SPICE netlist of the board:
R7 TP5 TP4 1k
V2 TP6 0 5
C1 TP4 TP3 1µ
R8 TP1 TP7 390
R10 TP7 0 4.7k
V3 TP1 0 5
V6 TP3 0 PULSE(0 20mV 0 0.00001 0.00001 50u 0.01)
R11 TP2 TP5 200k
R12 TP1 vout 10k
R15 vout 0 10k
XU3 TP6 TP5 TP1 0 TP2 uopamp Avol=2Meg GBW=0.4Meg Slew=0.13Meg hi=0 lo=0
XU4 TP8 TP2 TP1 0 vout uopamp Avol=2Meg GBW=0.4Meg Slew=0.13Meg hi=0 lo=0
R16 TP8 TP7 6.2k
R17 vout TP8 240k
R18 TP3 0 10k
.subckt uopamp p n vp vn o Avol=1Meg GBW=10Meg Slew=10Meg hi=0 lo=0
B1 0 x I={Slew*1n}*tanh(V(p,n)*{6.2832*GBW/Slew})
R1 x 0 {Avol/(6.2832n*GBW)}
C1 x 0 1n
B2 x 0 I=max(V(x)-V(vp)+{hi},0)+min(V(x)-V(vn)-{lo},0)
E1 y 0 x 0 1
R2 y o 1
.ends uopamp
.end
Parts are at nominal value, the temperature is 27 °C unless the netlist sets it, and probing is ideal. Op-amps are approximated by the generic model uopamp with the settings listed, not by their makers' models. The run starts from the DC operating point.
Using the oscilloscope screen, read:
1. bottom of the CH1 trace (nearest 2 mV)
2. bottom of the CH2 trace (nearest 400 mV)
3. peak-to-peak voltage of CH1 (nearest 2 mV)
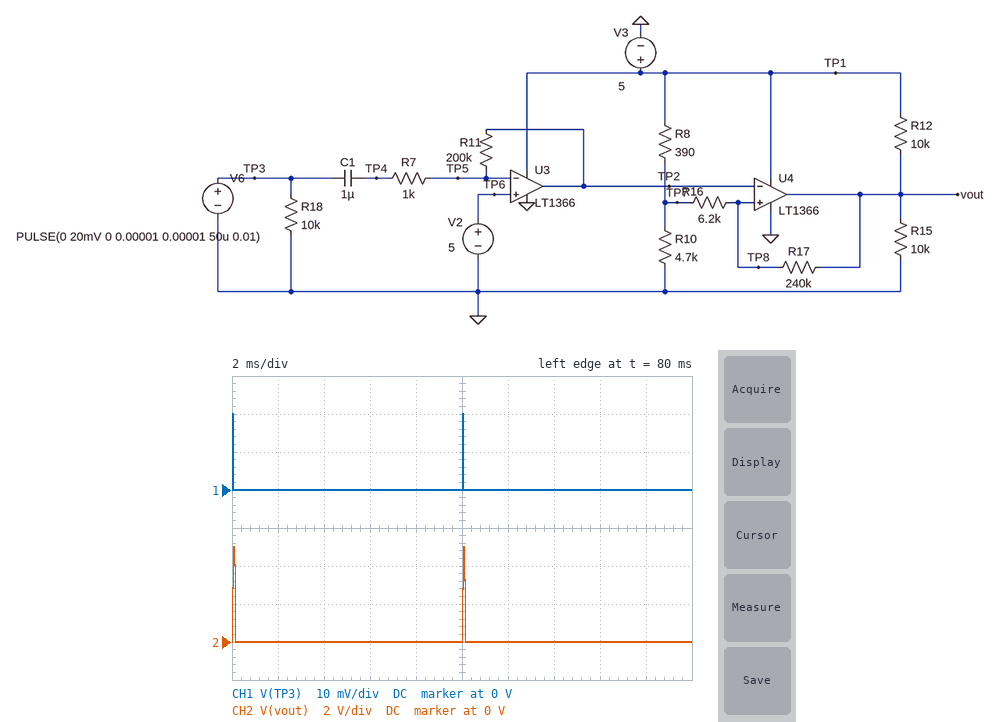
0 V
0 V
20 mV
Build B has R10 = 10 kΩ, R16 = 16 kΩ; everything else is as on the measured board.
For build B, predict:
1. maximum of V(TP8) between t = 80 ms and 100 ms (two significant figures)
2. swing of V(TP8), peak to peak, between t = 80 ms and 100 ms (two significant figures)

4.8 V
320 mV
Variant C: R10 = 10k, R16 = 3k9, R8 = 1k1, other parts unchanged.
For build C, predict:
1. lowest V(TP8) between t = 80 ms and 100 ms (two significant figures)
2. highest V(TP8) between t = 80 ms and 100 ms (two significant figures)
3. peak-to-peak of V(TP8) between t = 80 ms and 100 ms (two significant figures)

4.4 V
4.5 V
100 mV
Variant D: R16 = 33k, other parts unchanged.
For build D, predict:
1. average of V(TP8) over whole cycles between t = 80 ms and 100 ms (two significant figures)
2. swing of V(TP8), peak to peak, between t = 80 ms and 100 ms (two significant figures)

4.1 V
610 mV
